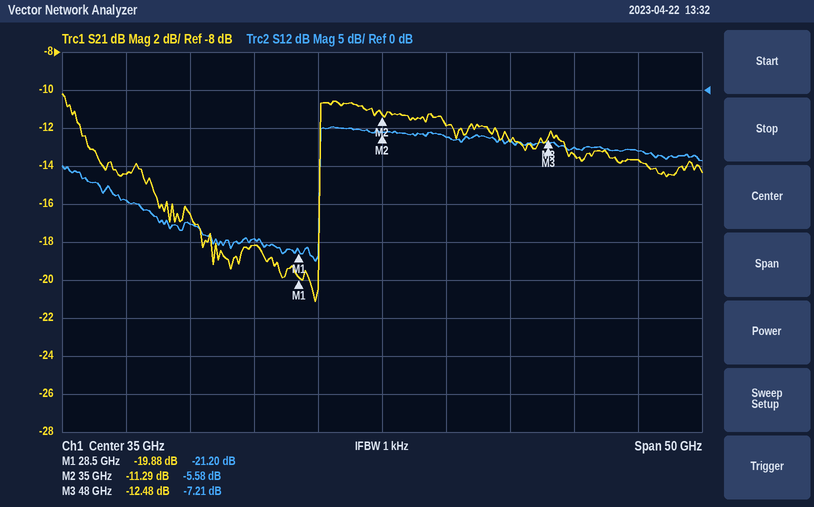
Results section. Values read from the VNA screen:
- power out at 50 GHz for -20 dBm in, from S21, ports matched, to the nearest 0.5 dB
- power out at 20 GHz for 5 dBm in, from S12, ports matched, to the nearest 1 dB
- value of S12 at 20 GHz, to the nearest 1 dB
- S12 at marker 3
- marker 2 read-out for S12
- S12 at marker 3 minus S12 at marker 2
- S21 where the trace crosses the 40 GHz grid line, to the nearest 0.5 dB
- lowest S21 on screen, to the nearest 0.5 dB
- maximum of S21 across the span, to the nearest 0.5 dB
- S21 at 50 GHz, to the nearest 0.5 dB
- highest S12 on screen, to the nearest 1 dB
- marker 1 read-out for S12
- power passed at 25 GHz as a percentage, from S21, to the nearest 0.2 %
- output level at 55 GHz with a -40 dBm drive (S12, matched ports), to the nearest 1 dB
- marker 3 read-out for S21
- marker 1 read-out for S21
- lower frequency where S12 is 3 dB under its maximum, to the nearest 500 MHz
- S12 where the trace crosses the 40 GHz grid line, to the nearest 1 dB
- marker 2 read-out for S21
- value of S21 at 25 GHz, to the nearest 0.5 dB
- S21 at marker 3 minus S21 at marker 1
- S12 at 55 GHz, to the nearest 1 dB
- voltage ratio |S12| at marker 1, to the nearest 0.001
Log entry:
-33.5 dBm
-13 dBm
-18 dB
-7.21 dB
-5.58 dB
-1.63 dB
-12.0 dB
-21.0 dB
-10.0 dB
-13.5 dB
-5 dB
-21.20 dB
1.6 %
-48 dBm
-12.48 dB
-19.88 dB
30.0 GHz
-6 dB
-11.29 dB
-18.0 dB
7.40 dB
-8 dB
0.087
